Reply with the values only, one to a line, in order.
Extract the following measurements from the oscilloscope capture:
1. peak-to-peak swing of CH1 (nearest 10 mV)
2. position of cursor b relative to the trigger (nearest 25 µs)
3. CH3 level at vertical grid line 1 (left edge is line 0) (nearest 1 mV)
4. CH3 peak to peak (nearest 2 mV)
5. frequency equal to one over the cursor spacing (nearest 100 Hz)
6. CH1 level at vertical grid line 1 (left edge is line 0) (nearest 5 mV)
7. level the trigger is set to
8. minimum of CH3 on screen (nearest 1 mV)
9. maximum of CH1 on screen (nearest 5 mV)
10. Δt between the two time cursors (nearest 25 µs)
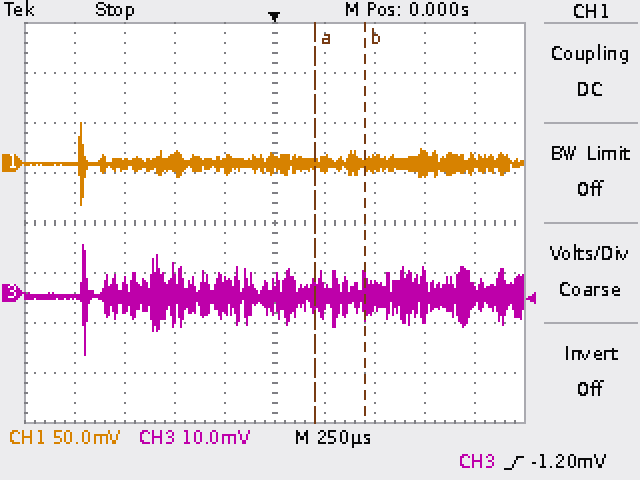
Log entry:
80 mV
+450 µs
-1 mV
22 mV
4.0 kHz
0 mV
-1.20 mV
-12 mV
40 mV
250 µs
